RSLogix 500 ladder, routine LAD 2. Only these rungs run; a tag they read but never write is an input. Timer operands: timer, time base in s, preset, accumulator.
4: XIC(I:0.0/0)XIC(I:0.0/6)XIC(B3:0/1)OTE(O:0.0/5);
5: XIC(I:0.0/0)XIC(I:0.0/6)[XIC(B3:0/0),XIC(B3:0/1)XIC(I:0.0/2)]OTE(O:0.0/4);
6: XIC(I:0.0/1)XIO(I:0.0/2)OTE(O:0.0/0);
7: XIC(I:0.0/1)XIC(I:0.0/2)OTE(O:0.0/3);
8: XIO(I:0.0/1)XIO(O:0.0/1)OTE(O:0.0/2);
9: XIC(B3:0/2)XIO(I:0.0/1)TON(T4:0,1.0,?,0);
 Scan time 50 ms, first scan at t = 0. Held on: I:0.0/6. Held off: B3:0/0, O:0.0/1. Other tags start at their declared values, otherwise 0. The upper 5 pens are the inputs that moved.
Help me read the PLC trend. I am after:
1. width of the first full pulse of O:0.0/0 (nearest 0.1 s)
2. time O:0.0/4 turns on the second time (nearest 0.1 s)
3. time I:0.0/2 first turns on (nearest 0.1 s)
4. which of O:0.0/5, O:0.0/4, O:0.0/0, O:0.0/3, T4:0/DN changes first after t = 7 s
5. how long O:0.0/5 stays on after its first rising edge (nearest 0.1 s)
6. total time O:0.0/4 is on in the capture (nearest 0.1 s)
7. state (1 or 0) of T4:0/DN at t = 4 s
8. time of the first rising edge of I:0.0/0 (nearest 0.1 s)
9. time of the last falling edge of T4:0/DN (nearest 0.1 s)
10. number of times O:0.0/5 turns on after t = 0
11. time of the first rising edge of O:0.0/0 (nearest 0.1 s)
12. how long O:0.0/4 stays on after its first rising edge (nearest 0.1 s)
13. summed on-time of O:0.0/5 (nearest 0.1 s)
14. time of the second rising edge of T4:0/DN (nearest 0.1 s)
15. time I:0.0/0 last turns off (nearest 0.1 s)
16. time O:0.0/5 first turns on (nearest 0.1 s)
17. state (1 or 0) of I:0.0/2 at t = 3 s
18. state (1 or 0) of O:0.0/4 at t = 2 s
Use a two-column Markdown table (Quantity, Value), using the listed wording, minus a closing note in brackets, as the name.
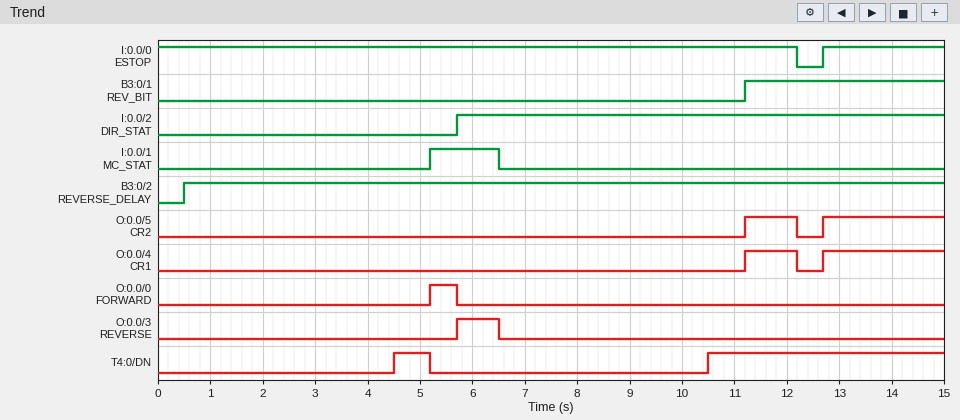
| Quantity | Value |
|---|---|
| width of the first full pulse of O:0.0/0 | 0.5 s |
| time O:0.0/4 turns on the second time | 12.7 s |
| time I:0.0/2 first turns on | 5.7 s |
| which of O:0.0/5, O:0.0/4, O:0.0/0, O:0.0/3, T4:0/DN changes first after t = 7 s | T4:0/DN |
| how long O:0.0/5 stays on after its first rising edge | 1.0 s |
| total time O:0.0/4 is on in the capture | 3.3 s |
| state (1 or 0) of T4:0/DN at t = 4 s | 0 |
| time of the first rising edge of I:0.0/0 | 12.7 s |
| time of the last falling edge of T4:0/DN | 5.2 s |
| number of times O:0.0/5 turns on after t = 0 | 2 |
| time of the first rising edge of O:0.0/0 | 5.2 s |
| how long O:0.0/4 stays on after its first rising edge | 1.0 s |
| summed on-time of O:0.0/5 | 3.3 s |
| time of the second rising edge of T4:0/DN | 10.5 s |
| time I:0.0/0 last turns off | 12.2 s |
| time O:0.0/5 first turns on | 11.2 s |
| state (1 or 0) of I:0.0/2 at t = 3 s | 0 |
| state (1 or 0) of O:0.0/4 at t = 2 s | 0 |
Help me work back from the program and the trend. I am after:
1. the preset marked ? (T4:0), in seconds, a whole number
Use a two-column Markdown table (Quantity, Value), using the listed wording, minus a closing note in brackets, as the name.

| Quantity | Value |
|---|---|
| the preset marked ? (T4:0), in seconds, a whole number | 4 s |
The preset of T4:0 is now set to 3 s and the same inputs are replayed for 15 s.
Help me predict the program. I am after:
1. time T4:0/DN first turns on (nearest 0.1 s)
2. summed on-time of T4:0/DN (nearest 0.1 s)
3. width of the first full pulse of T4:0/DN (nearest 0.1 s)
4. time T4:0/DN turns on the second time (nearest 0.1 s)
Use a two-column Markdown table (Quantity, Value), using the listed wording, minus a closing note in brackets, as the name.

| Quantity | Value |
|---|---|
| time T4:0/DN first turns on | 3.5 s |
| summed on-time of T4:0/DN | 7.2 s |
| width of the first full pulse of T4:0/DN | 1.7 s |
| time T4:0/DN turns on the second time | 9.5 s |
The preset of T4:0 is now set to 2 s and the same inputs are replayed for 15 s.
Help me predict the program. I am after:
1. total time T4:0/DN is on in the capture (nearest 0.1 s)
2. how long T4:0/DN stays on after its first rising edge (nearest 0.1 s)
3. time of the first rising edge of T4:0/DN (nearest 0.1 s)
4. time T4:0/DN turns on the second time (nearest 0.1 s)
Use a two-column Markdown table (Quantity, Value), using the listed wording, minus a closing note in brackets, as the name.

| Quantity | Value |
|---|---|
| total time T4:0/DN is on in the capture | 9.2 s |
| how long T4:0/DN stays on after its first rising edge | 2.7 s |
| time of the first rising edge of T4:0/DN | 2.5 s |
| time T4:0/DN turns on the second time | 8.5 s |
